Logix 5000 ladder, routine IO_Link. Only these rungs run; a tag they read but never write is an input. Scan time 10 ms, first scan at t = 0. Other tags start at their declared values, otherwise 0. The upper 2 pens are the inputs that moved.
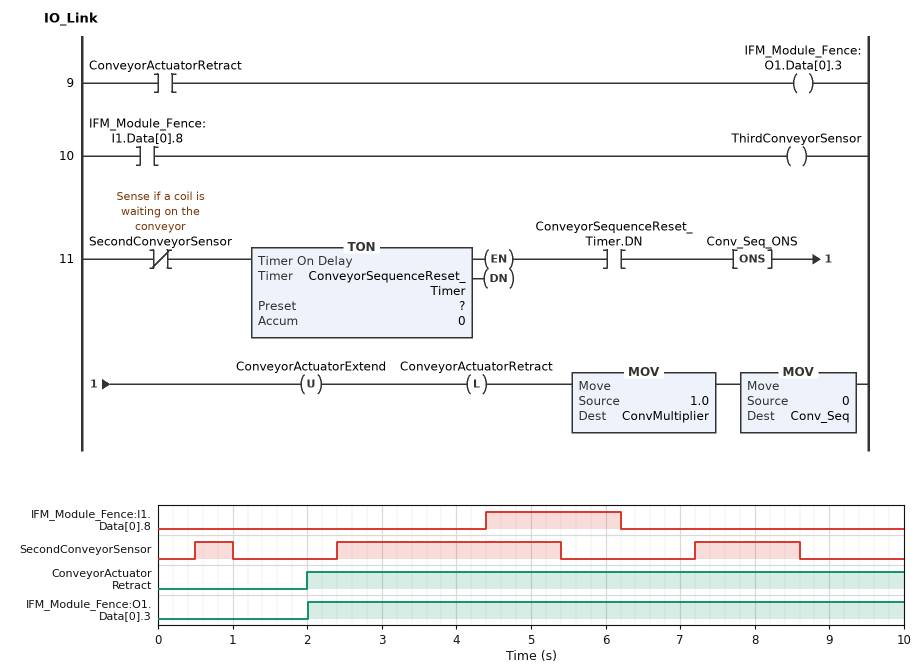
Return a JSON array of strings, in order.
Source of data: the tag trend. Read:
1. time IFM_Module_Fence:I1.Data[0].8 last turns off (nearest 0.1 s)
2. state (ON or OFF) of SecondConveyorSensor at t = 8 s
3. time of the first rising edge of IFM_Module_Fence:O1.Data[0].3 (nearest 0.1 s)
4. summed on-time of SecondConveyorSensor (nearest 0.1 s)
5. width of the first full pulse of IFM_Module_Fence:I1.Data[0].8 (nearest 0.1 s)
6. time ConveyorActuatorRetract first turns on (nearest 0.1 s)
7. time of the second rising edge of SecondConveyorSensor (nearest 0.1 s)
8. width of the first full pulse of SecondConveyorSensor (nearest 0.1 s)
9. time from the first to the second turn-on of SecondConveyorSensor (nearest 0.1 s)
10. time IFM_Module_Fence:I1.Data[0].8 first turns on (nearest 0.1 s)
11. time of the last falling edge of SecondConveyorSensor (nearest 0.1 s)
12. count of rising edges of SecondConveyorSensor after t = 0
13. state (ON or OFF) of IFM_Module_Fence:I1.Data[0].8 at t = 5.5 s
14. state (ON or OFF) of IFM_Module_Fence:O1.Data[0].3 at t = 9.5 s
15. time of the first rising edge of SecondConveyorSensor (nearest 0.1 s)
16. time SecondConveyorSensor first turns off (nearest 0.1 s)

["6.2 s", "ON", "2.0 s", "4.9 s", "1.8 s", "2.0 s", "2.4 s", "0.5 s", "1.9 s", "4.4 s", "8.6 s", "3", "ON", "ON", "0.5 s", "1.0 s"]
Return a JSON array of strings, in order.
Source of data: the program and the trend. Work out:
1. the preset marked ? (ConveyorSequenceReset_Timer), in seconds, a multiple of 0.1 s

["1.0 s"]
